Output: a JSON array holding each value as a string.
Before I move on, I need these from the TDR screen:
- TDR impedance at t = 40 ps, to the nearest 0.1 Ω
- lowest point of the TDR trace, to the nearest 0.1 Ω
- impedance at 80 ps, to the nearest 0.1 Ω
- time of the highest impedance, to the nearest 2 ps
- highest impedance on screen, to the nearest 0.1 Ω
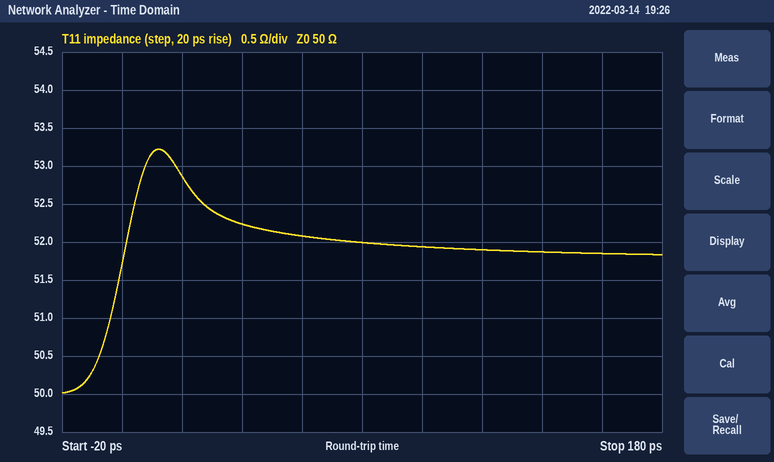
["52.2 Ω", "50.0 Ω", "52.0 Ω", "12 ps", "53.2 Ω"]
